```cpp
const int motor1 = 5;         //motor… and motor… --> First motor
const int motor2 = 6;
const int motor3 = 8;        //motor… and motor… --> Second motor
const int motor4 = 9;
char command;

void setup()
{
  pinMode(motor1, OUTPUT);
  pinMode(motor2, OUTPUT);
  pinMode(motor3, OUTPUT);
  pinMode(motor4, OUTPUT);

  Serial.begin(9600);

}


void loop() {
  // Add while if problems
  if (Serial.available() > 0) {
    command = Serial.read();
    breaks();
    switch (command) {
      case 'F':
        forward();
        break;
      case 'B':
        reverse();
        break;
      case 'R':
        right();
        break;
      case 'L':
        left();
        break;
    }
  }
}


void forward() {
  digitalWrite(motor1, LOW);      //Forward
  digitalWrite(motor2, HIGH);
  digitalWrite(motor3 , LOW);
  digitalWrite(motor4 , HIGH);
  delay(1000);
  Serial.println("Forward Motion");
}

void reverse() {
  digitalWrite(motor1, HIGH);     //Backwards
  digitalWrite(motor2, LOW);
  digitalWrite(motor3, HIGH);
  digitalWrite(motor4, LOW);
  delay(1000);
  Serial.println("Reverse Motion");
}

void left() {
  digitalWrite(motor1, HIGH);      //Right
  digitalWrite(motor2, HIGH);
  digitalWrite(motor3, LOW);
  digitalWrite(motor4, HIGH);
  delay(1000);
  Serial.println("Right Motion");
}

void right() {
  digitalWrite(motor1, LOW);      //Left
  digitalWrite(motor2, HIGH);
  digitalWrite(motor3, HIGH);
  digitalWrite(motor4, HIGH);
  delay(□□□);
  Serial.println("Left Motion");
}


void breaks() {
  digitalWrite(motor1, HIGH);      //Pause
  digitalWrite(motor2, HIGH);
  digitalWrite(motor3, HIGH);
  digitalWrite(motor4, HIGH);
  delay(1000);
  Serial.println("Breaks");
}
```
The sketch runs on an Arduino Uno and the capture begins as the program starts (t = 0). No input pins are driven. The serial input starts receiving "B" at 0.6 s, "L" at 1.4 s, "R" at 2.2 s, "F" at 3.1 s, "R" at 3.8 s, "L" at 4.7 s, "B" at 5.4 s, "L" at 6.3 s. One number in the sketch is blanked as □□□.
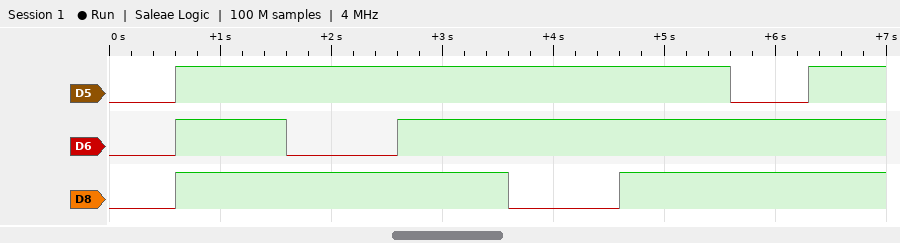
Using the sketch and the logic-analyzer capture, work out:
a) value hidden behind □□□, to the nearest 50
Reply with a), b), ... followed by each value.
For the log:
a) 700
